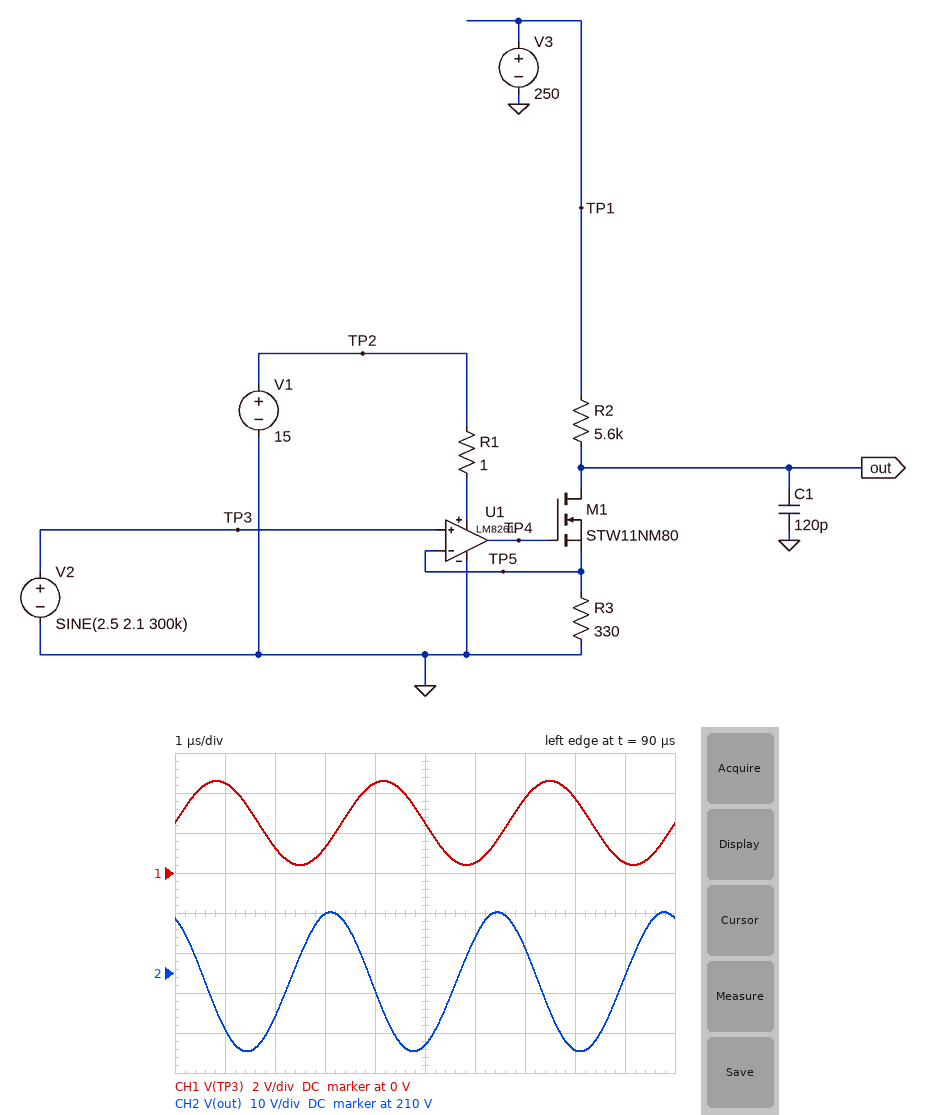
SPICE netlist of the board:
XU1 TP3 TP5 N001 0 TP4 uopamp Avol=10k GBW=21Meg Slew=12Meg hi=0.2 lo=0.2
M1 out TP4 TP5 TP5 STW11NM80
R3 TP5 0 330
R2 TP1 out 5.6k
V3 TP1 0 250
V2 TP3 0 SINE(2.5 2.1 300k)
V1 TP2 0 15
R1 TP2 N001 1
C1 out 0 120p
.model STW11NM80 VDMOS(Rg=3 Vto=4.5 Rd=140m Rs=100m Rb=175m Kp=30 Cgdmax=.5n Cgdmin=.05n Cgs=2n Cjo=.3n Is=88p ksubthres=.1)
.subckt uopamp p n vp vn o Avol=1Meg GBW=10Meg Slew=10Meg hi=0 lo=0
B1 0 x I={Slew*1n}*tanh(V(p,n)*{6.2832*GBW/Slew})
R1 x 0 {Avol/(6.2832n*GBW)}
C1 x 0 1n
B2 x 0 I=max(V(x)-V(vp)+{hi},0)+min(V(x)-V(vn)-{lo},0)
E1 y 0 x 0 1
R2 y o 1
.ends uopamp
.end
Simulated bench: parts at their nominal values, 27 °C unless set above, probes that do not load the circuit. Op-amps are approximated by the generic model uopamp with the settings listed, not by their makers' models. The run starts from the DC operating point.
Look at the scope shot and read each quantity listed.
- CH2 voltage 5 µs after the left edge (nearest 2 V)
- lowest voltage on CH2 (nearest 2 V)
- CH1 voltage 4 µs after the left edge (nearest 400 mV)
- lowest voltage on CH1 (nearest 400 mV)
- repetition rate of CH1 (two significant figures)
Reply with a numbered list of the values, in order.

1. 192 V
2. 190 V
3. 4.4 V
4. 400 mV
5. 300 kHz
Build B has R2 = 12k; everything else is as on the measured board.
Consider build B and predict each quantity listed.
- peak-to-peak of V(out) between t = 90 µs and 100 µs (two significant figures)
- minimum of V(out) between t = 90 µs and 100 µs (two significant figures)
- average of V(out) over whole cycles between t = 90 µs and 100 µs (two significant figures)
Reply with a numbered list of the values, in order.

1. 38 V
2. 140 V
3. 160 V
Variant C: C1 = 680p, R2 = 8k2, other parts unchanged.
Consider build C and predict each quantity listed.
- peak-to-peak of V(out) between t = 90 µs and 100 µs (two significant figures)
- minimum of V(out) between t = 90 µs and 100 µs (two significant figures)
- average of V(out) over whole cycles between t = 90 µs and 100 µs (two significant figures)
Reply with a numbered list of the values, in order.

1. 9.2 V
2. 180 V
3. 190 V
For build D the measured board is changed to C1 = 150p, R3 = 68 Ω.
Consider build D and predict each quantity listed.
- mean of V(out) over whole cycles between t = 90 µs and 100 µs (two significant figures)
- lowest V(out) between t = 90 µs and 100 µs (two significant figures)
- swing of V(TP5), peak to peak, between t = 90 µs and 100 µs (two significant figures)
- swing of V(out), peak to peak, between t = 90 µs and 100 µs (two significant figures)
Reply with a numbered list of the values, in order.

1. 44 V
2. 1.4 V
3. 4.2 V
4. 110 V
